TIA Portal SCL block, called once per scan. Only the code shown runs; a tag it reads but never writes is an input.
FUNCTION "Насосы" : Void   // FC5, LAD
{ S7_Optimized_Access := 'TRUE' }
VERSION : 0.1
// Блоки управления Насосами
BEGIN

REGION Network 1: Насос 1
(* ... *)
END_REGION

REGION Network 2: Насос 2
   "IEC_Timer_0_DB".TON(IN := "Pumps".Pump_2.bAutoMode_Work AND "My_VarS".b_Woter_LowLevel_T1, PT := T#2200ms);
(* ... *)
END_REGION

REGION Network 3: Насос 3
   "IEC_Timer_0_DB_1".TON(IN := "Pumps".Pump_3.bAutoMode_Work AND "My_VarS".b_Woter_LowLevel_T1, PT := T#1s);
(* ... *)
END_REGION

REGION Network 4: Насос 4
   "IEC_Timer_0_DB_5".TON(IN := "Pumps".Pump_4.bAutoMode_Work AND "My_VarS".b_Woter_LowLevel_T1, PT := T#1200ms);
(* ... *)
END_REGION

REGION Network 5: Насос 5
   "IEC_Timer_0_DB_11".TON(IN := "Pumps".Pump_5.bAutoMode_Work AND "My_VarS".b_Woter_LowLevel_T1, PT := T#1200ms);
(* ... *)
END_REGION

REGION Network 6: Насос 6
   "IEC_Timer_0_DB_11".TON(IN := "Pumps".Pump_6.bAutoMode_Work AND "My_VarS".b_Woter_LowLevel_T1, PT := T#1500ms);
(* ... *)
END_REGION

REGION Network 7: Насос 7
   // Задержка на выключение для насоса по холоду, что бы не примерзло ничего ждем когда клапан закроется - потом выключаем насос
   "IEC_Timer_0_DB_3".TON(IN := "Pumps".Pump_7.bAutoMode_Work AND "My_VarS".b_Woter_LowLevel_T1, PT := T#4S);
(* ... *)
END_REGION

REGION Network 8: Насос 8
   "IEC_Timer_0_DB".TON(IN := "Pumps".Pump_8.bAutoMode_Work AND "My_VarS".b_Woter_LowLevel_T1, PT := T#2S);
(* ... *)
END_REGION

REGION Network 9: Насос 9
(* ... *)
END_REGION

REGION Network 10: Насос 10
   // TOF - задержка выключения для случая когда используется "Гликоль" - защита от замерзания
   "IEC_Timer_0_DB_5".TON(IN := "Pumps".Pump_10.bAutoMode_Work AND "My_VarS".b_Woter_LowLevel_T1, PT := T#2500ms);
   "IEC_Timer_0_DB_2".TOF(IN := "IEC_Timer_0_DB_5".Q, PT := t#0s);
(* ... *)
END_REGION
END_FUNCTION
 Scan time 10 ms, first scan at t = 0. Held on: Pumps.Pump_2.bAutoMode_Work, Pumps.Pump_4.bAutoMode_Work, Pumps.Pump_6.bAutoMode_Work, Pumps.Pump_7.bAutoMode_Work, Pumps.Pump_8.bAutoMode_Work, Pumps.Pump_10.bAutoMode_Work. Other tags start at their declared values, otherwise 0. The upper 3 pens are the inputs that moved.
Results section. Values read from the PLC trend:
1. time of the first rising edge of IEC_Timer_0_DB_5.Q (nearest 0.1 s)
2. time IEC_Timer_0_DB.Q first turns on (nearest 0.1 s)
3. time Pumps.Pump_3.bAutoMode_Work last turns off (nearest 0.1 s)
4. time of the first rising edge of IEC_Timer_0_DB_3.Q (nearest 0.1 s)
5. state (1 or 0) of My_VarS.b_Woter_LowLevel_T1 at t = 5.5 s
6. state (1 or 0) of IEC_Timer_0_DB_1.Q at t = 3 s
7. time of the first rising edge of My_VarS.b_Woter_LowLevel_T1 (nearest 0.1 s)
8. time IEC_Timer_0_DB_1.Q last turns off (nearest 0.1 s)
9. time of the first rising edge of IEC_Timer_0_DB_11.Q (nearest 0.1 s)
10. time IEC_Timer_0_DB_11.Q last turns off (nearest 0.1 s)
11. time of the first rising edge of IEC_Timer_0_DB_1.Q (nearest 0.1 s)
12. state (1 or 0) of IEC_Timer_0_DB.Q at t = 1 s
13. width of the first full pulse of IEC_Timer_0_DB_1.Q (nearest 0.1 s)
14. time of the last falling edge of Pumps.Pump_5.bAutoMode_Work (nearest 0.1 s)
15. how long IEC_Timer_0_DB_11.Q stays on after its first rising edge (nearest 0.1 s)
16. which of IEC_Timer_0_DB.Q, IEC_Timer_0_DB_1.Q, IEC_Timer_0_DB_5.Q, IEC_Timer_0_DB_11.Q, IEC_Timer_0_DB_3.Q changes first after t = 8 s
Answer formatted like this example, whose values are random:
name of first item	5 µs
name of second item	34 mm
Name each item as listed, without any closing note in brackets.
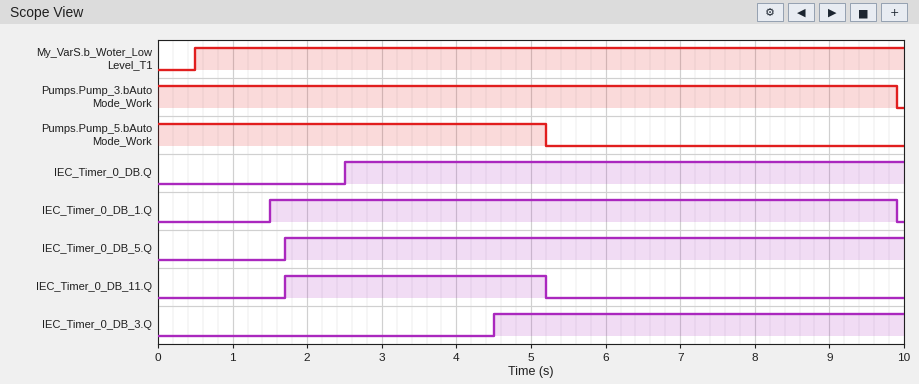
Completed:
time of the first rising edge of IEC_Timer_0_DB_5.Q	1.7 s
time IEC_Timer_0_DB.Q first turns on	2.5 s
time Pumps.Pump_3.bAutoMode_Work last turns off	9.9 s
time of the first rising edge of IEC_Timer_0_DB_3.Q	4.5 s
state (1 or 0) of My_VarS.b_Woter_LowLevel_T1 at t = 5.5 s	1
state (1 or 0) of IEC_Timer_0_DB_1.Q at t = 3 s	1
time of the first rising edge of My_VarS.b_Woter_LowLevel_T1	0.5 s
time IEC_Timer_0_DB_1.Q last turns off	9.9 s
time of the first rising edge of IEC_Timer_0_DB_11.Q	1.7 s
time IEC_Timer_0_DB_11.Q last turns off	5.2 s
time of the first rising edge of IEC_Timer_0_DB_1.Q	1.5 s
state (1 or 0) of IEC_Timer_0_DB.Q at t = 1 s	0
width of the first full pulse of IEC_Timer_0_DB_1.Q	8.4 s
time of the last falling edge of Pumps.Pump_5.bAutoMode_Work	5.2 s
how long IEC_Timer_0_DB_11.Q stays on after its first rising edge	3.5 s
which of IEC_Timer_0_DB.Q, IEC_Timer_0_DB_1.Q, IEC_Timer_0_DB_5.Q, IEC_Timer_0_DB_11.Q, IEC_Timer_0_DB_3.Q changes first after t = 8 s	IEC_Timer_0_DB_1.Q
